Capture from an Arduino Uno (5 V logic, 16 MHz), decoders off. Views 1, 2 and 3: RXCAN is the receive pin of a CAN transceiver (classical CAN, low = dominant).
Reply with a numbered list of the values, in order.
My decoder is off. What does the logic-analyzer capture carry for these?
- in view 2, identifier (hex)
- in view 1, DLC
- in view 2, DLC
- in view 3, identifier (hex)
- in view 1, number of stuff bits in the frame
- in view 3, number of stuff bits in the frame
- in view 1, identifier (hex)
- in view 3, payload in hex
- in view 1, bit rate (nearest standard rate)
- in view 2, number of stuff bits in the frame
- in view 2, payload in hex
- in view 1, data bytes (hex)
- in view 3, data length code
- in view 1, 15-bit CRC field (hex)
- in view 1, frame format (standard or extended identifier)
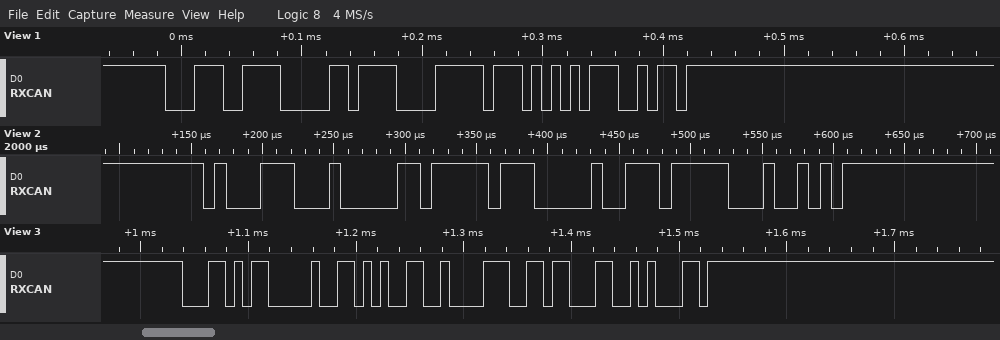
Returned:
1. 0x471
2. 2
3. 2
4. 0x1AC
5. 2
6. 1
7. 0x1CF
8. 53 21 CD
9. 125 kbit/s
10. 4
11. FF 01
12. F0 FF
13. 3
14. 0x2AE5
15. standard
